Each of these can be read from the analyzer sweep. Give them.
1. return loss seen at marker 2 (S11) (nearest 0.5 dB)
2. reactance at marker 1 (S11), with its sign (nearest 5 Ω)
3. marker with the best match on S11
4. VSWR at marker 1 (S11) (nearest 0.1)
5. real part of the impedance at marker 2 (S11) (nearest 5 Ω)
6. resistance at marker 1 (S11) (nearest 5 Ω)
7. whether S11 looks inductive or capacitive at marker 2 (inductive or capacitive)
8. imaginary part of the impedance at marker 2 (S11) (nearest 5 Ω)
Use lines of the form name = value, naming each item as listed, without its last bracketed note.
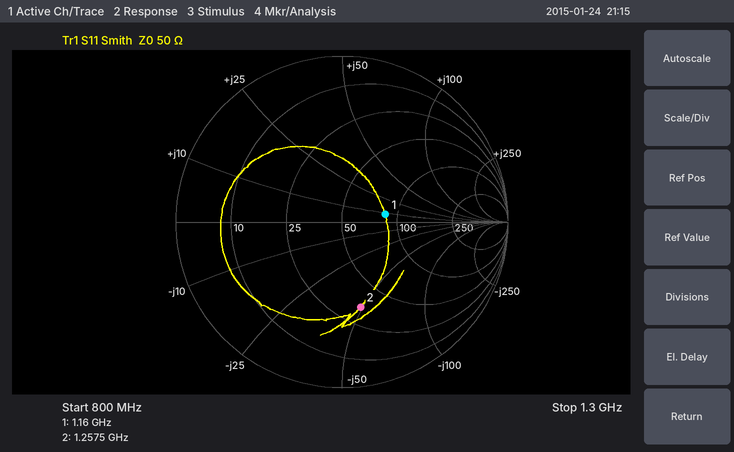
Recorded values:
return loss seen at marker 2 (S11) = 5.5 dB
reactance at marker 1 (S11), with its sign = +10 Ω
marker with the best match on S11 = marker 1
VSWR at marker 1 (S11) = 1.7
real part of the impedance at marker 2 (S11) = 35 Ω
resistance at marker 1 (S11) = 85 Ω
whether S11 looks inductive or capacitive at marker 2 = capacitive
imaginary part of the impedance at marker 2 (S11) = -50 Ω
